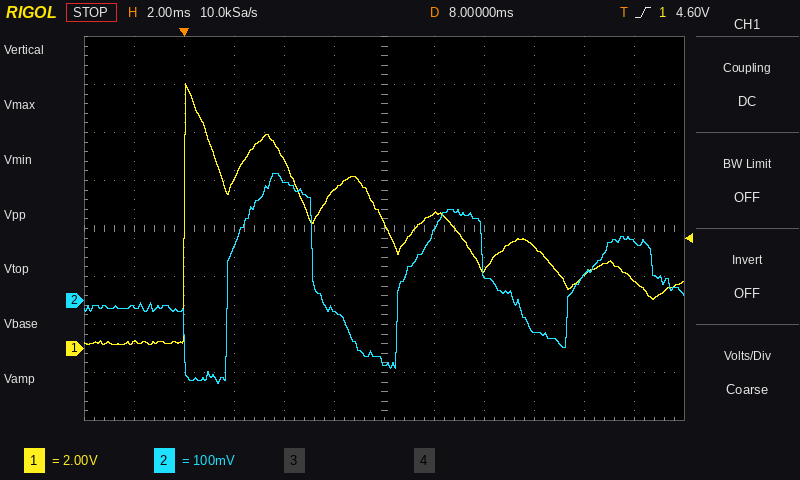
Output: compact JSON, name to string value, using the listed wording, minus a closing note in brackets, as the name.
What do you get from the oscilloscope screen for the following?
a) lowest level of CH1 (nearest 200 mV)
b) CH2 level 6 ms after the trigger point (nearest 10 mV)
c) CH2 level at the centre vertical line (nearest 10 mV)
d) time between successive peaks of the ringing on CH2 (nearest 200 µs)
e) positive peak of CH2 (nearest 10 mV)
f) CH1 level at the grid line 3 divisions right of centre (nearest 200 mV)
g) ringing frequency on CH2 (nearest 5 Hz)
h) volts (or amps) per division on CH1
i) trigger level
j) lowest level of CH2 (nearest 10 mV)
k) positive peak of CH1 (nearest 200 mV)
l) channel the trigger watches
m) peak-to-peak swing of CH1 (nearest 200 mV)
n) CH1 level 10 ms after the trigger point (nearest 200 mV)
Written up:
{"lowest level of CH1": "200 mV", "CH2 level 6 ms after the trigger point": "-20 mV", "CH2 level at the centre vertical line": "-130 mV", "time between successive peaks of the ringing on CH2": "7.0 ms", "positive peak of CH2": "260 mV", "CH1 level at the grid line 3 divisions right of centre": "4.2 V", "ringing frequency on CH2": "145 Hz", "volts (or amps) per division on CH1": "2 V", "trigger level": "4.60 V", "lowest level of CH2": "-170 mV", "positive peak of CH1": "11.0 V", "channel the trigger watches": "CH1", "peak-to-peak swing of CH1": "10.8 V", "CH1 level 10 ms after the trigger point": "5.6 V"}
